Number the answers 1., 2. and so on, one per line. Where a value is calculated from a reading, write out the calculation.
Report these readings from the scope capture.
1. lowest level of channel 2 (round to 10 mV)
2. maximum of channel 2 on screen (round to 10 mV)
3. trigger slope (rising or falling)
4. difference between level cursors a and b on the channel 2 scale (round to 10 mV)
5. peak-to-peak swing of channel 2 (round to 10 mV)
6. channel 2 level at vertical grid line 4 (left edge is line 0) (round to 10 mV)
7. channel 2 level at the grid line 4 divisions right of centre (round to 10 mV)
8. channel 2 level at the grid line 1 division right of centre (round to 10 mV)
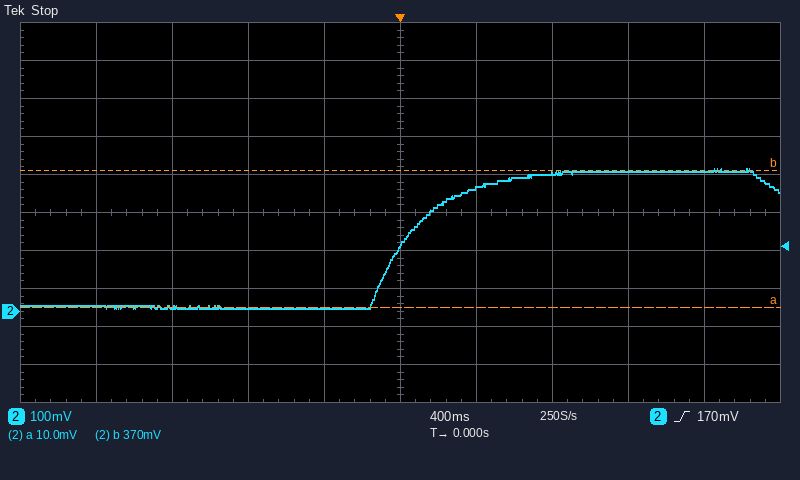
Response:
1. 10 mV
2. 380 mV
3. rising
4. 360 mV
5. 380 mV − (10 mV) = 370 mV
6. 10 mV
7. 370 mV
8. 320 mV
